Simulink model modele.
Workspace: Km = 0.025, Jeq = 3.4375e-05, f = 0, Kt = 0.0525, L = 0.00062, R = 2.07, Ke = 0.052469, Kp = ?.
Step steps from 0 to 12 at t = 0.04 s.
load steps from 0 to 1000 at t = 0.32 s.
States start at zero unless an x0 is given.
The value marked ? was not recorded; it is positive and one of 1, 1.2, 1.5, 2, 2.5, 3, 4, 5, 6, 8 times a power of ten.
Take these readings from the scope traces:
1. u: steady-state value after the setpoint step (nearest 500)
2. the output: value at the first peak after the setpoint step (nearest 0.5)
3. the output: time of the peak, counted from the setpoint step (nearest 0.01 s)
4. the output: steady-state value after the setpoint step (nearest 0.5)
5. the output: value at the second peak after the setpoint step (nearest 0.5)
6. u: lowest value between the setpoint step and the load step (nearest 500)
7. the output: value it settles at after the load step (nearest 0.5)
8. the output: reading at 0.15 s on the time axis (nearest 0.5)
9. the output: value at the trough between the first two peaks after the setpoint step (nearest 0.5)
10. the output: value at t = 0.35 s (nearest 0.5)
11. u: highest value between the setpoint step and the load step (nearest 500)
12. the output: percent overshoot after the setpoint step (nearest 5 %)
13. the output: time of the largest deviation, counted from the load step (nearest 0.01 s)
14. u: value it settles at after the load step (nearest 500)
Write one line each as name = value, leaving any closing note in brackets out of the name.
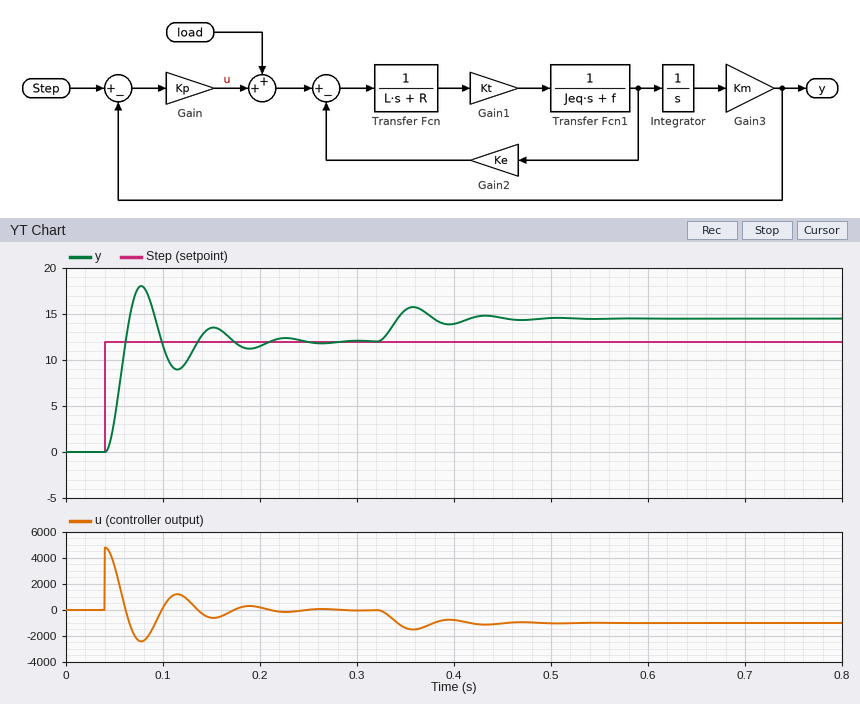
u: steady-state value after the setpoint step = 0
the output: value at the first peak after the setpoint step = 18.0
the output: time of the peak, counted from the setpoint step = 0.04 s
the output: steady-state value after the setpoint step = 12.0
the output: value at the second peak after the setpoint step = 13.5
u: lowest value between the setpoint step and the load step = -2500
the output: value it settles at after the load step = 14.5
the output: reading at 0.15 s on the time axis = 13.5
the output: value at the trough between the first two peaks after the setpoint step = 9.0
the output: value at t = 0.35 s = 15.5
u: highest value between the setpoint step and the load step = 5000
the output: percent overshoot after the setpoint step = 50 %
the output: time of the largest deviation, counted from the load step = 0.04 s
u: value it settles at after the load step = -1000
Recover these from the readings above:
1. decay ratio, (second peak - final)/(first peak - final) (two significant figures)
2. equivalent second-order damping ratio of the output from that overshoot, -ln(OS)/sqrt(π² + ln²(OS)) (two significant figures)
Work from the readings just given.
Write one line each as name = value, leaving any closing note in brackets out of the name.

decay ratio, (second peak - final)/(first peak - final) = 0.25
equivalent second-order damping ratio of the output from that overshoot, -ln(OS)/sqrt(π² + ln²(OS)) = 0.22
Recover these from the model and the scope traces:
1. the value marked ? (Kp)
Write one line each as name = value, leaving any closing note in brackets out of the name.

the value marked ? = 400
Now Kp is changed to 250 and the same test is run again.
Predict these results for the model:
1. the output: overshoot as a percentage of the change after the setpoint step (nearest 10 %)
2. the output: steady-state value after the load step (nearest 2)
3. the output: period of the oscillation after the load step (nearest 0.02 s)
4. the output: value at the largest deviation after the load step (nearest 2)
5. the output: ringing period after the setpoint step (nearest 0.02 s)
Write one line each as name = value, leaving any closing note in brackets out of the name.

the output: overshoot as a percentage of the change after the setpoint step = 40 %
the output: steady-state value after the load step = 16
the output: period of the oscillation after the load step = 0.10 s
the output: value at the largest deviation after the load step = 18
the output: ringing period after the setpoint step = 0.10 s
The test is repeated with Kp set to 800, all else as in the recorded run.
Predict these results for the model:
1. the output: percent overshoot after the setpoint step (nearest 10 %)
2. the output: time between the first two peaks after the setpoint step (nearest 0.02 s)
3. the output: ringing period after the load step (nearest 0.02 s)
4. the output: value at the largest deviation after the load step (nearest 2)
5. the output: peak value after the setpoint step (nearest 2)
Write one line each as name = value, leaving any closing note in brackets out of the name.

the output: percent overshoot after the setpoint step = 60 %
the output: time between the first two peaks after the setpoint step = 0.06 s
the output: ringing period after the load step = 0.06 s
the output: value at the largest deviation after the load step = 14
the output: peak value after the setpoint step = 20
